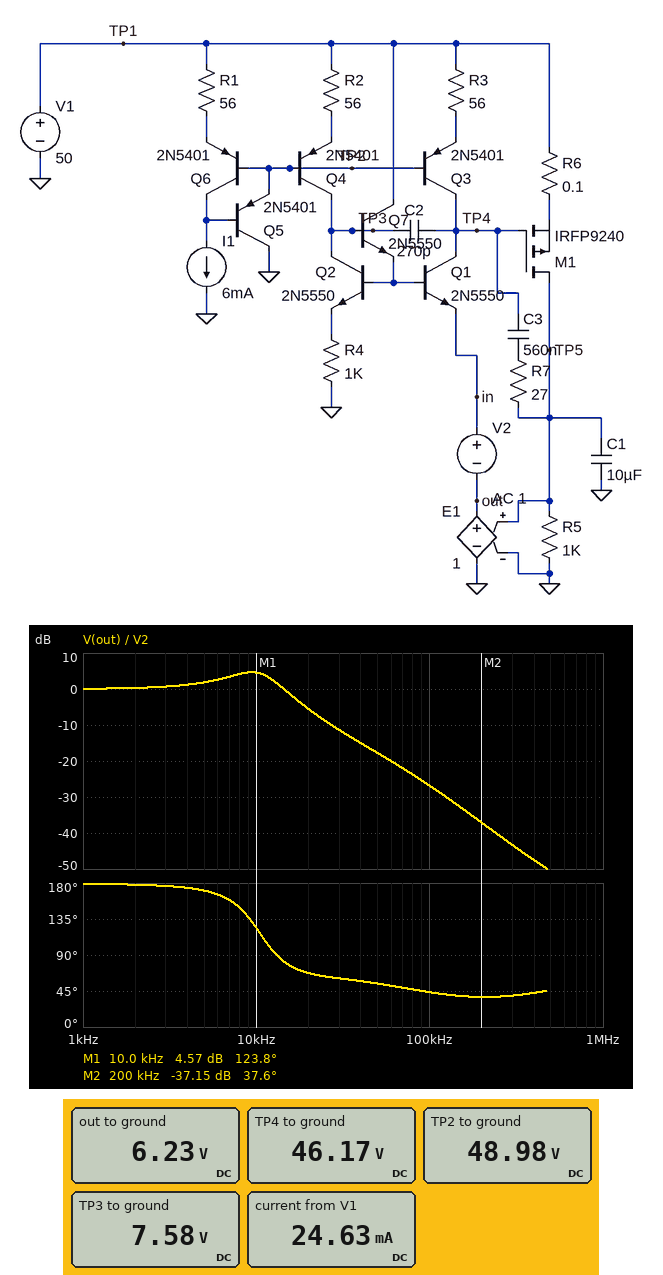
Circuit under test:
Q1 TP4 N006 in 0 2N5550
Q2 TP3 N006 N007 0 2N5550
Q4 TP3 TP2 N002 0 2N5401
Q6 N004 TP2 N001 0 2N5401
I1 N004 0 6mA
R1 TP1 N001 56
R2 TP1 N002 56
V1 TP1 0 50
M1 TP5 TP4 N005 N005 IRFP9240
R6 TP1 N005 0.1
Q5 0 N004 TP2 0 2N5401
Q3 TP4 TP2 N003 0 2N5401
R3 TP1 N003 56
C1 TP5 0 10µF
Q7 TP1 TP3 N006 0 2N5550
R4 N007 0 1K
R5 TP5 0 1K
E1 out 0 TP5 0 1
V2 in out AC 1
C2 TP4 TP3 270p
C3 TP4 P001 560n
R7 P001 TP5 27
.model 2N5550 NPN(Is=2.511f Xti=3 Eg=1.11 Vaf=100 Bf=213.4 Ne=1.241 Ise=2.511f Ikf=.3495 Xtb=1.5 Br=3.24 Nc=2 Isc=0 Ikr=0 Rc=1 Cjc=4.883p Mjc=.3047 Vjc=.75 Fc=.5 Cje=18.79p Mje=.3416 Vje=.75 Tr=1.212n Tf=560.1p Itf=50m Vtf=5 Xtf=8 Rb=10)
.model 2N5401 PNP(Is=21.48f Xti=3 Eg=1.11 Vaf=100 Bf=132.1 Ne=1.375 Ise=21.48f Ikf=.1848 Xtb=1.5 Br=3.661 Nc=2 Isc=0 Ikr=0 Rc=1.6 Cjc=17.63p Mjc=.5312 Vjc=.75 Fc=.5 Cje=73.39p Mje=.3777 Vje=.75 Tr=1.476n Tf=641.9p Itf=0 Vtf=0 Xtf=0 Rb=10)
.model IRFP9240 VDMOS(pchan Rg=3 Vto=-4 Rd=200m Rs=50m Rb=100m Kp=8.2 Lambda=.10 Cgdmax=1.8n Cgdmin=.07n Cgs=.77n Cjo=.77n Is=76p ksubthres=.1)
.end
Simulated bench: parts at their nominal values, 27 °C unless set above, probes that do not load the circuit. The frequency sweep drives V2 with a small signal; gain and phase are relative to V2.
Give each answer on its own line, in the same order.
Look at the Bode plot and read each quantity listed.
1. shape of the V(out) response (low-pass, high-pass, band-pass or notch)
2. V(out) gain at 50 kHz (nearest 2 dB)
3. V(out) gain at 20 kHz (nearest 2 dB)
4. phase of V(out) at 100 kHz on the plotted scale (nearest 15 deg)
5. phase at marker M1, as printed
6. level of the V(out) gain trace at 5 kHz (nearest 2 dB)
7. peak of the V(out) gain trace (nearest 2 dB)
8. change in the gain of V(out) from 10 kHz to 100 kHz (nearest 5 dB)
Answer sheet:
low-pass
-18 dB
-6 dB
45 deg
123.8 deg
2 dB
4 dB
-30 dB
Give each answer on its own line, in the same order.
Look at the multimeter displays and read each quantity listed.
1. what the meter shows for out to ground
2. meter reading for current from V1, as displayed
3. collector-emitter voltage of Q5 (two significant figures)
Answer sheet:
6.23 V
24.63 mA
-49 V
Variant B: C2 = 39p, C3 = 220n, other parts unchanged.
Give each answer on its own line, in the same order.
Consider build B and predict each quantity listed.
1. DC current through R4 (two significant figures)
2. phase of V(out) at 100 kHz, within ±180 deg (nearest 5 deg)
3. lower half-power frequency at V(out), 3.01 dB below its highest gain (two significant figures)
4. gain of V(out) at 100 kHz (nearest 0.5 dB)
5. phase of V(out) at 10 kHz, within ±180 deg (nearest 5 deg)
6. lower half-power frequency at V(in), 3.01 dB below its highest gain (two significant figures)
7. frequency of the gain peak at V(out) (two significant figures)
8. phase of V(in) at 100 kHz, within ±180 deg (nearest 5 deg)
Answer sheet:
6.2 mA
65 deg
11 kHz
-22.5 dB
170 deg
14 kHz
16 kHz
5 deg
